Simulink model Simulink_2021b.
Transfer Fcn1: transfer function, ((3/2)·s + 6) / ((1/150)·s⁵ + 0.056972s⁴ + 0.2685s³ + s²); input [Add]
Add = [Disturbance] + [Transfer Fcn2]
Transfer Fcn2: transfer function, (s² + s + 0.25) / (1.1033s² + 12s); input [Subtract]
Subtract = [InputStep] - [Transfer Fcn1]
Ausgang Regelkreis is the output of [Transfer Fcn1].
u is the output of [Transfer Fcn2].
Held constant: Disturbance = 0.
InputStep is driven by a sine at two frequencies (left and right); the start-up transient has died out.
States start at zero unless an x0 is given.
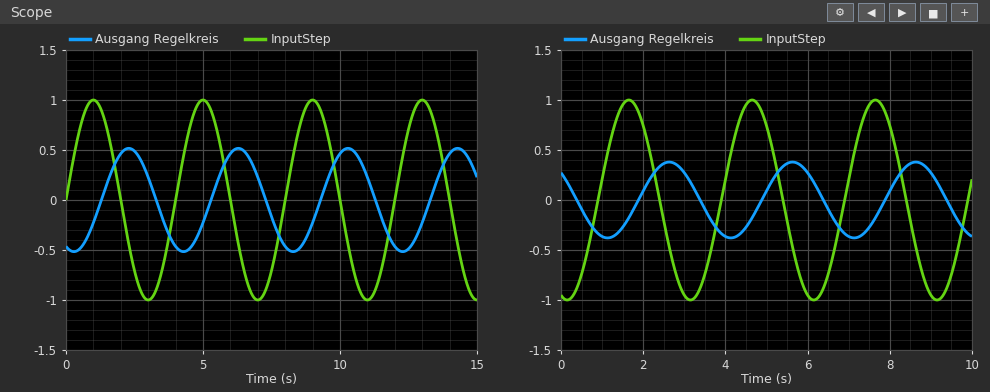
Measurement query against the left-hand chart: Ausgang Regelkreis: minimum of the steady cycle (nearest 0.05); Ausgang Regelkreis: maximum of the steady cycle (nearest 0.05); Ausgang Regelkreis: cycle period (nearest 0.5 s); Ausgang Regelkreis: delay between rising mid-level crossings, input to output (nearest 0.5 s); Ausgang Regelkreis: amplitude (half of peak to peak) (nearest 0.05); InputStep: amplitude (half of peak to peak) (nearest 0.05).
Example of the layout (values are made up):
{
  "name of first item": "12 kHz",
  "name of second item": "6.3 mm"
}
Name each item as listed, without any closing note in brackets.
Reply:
{
  "Ausgang Regelkreis: minimum of the steady cycle": "-0.50",
  "Ausgang Regelkreis: maximum of the steady cycle": "0.50",
  "Ausgang Regelkreis: cycle period": "4.0 s",
  "Ausgang Regelkreis: delay between rising mid-level crossings, input to output": "1.5 s",
  "Ausgang Regelkreis: amplitude (half of peak to peak)": "0.50",
  "InputStep: amplitude (half of peak to peak)": "1.00"
}
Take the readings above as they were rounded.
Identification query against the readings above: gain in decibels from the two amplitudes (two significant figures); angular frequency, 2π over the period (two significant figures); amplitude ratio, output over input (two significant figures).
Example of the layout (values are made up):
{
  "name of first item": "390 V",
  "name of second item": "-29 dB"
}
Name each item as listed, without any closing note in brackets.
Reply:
{
  "gain in decibels from the two amplitudes": "-6.0 dB",
  "angular frequency, 2π over the period": "1.6 rad/s",
  "amplitude ratio, output over input": "0.50"
}
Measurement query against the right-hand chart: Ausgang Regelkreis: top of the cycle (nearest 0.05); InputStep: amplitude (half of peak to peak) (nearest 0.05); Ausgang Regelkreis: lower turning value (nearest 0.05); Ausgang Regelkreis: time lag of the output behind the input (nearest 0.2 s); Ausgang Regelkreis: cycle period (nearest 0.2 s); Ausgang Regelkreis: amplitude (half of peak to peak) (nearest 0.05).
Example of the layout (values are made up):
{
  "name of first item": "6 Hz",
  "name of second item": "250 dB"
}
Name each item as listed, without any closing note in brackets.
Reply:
{
  "Ausgang Regelkreis: top of the cycle": "0.40",
  "InputStep: amplitude (half of peak to peak)": "1.00",
  "Ausgang Regelkreis: lower turning value": "-0.40",
  "Ausgang Regelkreis: time lag of the output behind the input": "1.0 s",
  "Ausgang Regelkreis: cycle period": "3.0 s",
  "Ausgang Regelkreis: amplitude (half of peak to peak)": "0.40"
}
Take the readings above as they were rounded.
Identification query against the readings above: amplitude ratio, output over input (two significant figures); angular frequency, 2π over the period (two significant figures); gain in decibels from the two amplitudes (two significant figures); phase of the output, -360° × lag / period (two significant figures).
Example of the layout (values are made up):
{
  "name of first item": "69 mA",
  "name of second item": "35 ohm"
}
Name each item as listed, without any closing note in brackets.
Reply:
{
  "amplitude ratio, output over input": "0.40",
  "angular frequency, 2π over the period": "2.1 rad/s",
  "gain in decibels from the two amplitudes": "-8.0 dB",
  "phase of the output, -360° × lag / period": "-120°"
}
